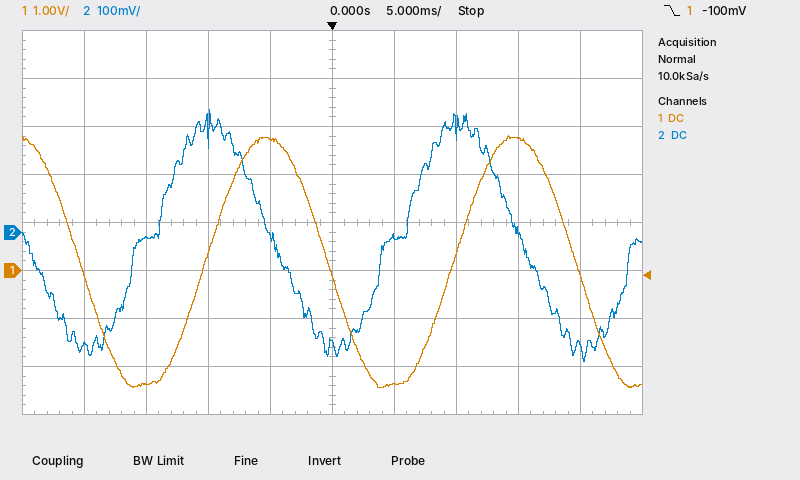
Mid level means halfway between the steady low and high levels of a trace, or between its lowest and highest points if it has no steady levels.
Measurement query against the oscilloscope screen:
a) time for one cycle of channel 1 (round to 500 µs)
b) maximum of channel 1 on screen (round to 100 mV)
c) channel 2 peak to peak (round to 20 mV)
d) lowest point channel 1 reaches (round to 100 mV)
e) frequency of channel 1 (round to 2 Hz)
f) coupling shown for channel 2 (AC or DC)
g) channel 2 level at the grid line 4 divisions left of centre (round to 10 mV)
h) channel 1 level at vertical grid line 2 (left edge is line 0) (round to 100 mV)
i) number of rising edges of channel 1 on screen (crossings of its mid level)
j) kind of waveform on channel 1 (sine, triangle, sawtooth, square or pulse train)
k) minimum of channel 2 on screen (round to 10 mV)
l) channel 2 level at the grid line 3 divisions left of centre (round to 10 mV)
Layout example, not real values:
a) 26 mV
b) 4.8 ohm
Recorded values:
a) 20.0 ms
b) 2.8 V
c) 520 mV
d) -2.4 V
e) 50 Hz
f) DC
g) -240 mV
h) -2.4 V
i) 2
j) sine
k) -270 mV
l) -10 mV
